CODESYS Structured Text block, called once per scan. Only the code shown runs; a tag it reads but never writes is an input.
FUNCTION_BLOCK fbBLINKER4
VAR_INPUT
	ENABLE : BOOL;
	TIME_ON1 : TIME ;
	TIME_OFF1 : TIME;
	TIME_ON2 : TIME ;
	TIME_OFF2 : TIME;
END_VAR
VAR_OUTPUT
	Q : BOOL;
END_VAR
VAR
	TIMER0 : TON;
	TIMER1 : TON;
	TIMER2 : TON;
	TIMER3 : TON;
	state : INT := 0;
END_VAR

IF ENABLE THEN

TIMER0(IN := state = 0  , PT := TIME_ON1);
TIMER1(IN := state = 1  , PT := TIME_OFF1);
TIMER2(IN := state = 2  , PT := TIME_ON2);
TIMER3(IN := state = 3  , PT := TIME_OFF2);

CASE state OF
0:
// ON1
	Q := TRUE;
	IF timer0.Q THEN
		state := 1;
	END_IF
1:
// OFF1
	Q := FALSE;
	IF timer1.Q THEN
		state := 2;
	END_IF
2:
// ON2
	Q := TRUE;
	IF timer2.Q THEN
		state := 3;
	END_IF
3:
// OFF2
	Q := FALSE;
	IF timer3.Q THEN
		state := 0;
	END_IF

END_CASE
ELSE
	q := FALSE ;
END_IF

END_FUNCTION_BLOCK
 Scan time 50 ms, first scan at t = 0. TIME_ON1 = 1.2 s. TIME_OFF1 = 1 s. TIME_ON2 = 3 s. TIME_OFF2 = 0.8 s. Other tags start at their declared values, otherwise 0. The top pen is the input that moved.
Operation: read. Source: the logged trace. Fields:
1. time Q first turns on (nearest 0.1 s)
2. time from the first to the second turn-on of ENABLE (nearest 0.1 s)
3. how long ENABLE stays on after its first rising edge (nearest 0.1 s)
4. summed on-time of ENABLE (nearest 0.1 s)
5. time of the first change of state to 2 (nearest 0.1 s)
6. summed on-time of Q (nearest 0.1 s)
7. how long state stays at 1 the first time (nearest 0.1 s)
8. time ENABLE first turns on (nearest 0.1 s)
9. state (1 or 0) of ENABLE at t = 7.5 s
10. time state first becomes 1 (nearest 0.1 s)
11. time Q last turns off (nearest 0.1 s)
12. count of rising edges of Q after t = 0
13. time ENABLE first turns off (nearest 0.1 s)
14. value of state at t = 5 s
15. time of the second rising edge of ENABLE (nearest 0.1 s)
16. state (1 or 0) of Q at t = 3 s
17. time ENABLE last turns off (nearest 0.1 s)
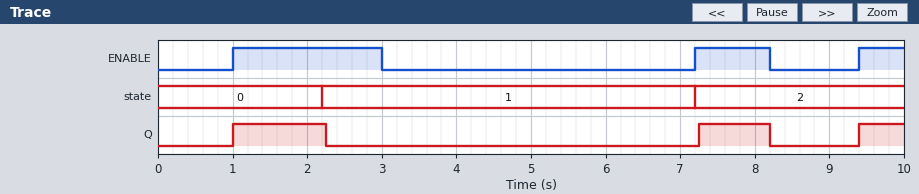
1.0 s
6.2 s
2.0 s
3.6 s
7.2 s
2.8 s
5.0 s
1.0 s
1
2.2 s
8.2 s
3
3.0 s
1
7.2 s
0
8.2 s
